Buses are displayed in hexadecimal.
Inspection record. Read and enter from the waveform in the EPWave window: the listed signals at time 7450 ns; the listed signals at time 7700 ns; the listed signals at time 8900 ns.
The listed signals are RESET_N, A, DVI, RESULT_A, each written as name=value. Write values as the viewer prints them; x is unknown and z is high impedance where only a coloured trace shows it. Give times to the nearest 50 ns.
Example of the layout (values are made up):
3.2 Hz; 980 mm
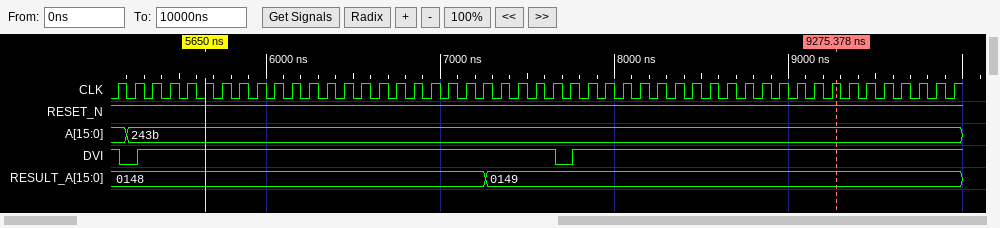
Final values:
RESET_N=1, A=243b, DVI=1, RESULT_A=0149; RESET_N=1, A=243b, DVI=0, RESULT_A=0149; RESET_N=1, A=243b, DVI=1, RESULT_A=0149
